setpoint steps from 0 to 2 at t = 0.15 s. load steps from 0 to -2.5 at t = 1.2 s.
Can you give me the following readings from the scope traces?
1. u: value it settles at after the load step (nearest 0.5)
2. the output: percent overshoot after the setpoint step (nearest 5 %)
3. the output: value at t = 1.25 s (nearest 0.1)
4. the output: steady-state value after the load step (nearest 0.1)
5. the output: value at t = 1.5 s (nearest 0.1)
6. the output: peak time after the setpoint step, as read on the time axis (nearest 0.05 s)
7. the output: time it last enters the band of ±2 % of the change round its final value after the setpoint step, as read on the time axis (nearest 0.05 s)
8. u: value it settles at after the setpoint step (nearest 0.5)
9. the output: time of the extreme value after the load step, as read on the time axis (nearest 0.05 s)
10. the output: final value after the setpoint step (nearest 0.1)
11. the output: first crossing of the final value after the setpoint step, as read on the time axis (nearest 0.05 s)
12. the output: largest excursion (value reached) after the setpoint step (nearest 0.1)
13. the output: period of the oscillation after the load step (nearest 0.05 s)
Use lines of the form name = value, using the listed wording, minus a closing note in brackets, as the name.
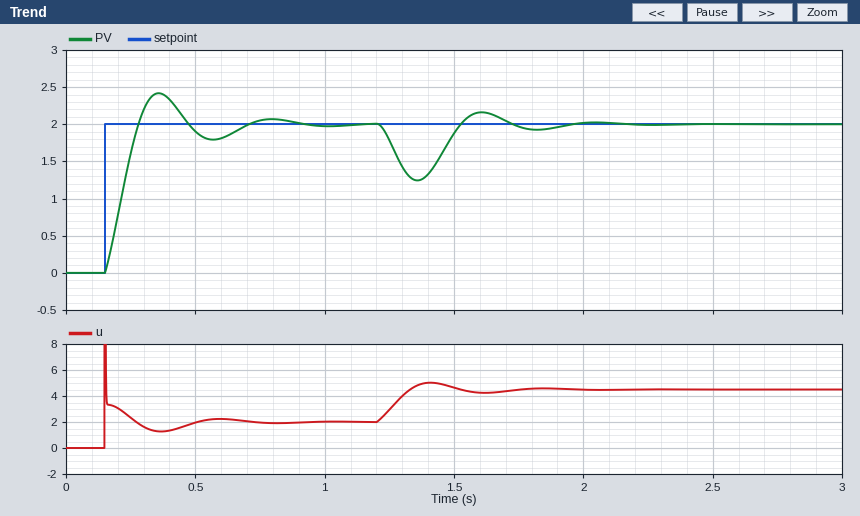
u: value it settles at after the load step = 4.5
the output: percent overshoot after the setpoint step = 20 %
the output: value at t = 1.25 s = 1.8
the output: steady-state value after the load step = 2.0
the output: value at t = 1.5 s = 1.9
the output: peak time after the setpoint step, as read on the time axis = 0.35 s
the output: time it last enters the band of ±2 % of the change round its final value after the setpoint step, as read on the time axis = 0.85 s
u: value it settles at after the setpoint step = 2.0
the output: time of the extreme value after the load step, as read on the time axis = 1.35 s
the output: final value after the setpoint step = 2.0
the output: first crossing of the final value after the setpoint step, as read on the time axis = 0.30 s
the output: largest excursion (value reached) after the setpoint step = 2.4
the output: period of the oscillation after the load step = 0.45 s
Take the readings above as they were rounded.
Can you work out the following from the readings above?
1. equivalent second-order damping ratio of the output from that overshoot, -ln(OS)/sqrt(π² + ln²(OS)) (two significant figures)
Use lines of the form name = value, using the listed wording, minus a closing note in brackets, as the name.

equivalent second-order damping ratio of the output from that overshoot, -ln(OS)/sqrt(π² + ln²(OS)) = 0.46
